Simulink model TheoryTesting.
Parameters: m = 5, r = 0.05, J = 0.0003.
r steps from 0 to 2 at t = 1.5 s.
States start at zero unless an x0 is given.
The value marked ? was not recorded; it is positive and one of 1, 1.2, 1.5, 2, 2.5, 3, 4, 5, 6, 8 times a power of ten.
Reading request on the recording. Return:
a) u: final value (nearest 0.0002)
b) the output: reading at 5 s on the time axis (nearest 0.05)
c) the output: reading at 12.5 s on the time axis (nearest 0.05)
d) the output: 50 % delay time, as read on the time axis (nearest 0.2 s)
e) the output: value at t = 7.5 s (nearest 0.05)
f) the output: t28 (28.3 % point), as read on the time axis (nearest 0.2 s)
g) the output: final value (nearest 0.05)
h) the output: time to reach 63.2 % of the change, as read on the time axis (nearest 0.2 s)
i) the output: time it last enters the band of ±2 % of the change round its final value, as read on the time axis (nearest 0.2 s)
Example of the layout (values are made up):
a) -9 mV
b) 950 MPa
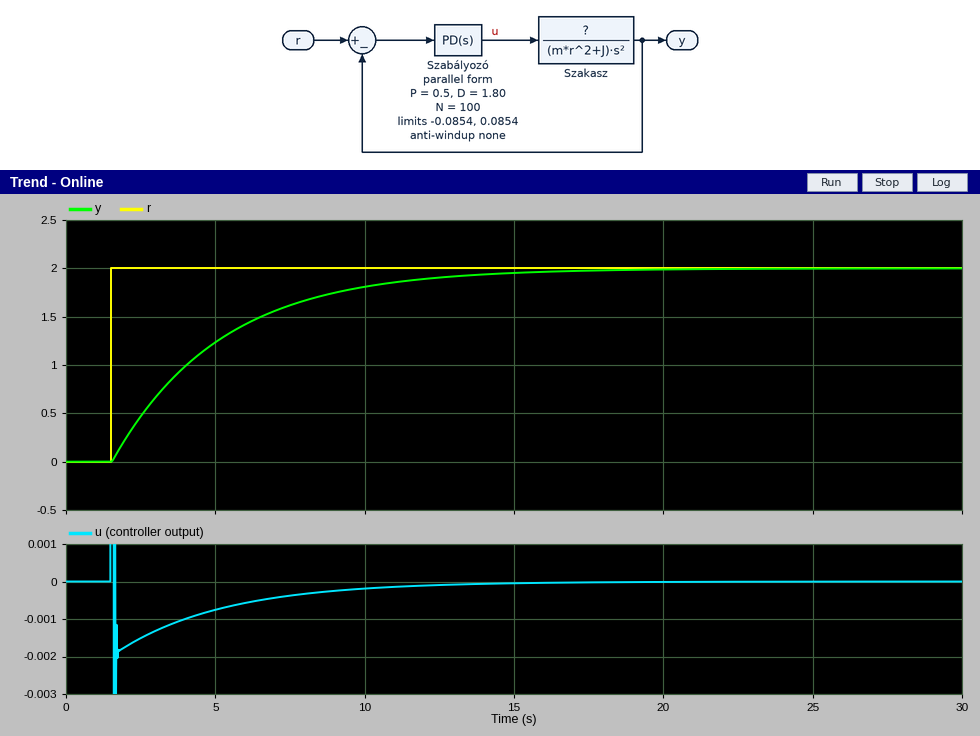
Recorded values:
a) 0.0000
b) 1.25
c) 1.90
d) 4.0 s
e) 1.60
f) 2.8 s
g) 2.00
h) 5.2 s
i) 15.6 s
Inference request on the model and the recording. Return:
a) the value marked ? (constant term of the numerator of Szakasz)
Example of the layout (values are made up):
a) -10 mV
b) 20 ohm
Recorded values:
a) 1
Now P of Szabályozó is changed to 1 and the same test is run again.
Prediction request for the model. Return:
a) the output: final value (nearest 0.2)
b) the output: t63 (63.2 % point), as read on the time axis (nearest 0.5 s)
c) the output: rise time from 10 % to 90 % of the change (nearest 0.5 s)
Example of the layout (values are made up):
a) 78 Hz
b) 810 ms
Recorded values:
a) 2.0
b) 3.5 s
c) 4.0 s
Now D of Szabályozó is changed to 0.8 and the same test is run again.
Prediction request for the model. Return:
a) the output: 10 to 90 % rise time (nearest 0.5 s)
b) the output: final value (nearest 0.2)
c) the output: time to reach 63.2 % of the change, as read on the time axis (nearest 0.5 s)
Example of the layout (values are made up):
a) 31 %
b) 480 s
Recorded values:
a) 3.5 s
b) 2.0
c) 3.0 s
